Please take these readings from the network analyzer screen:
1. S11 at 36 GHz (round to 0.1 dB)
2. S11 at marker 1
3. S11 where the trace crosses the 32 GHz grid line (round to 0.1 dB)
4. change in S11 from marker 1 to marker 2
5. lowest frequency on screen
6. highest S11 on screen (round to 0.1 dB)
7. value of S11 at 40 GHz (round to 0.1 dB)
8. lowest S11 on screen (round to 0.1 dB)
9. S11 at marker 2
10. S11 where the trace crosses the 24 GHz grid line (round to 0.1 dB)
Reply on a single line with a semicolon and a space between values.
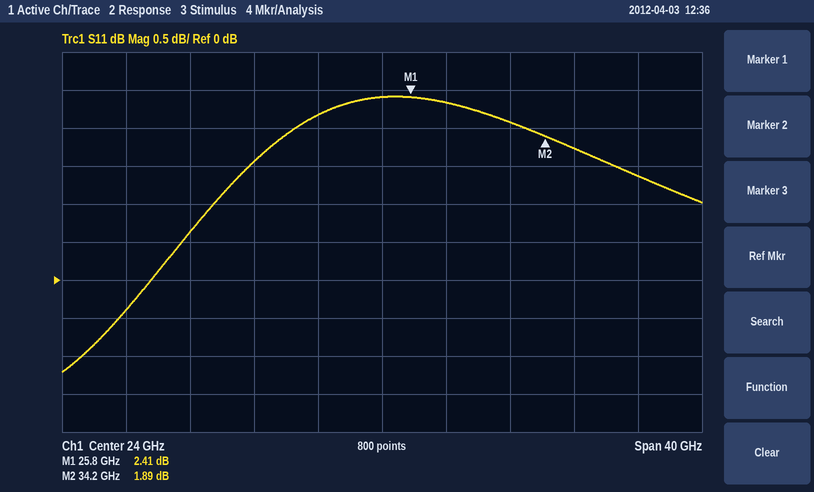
1.7 dB; 2.41 dB; 2.1 dB; -0.52 dB; 4 GHz; 2.4 dB; 1.4 dB; -1.2 dB; 1.89 dB; 2.4 dB
